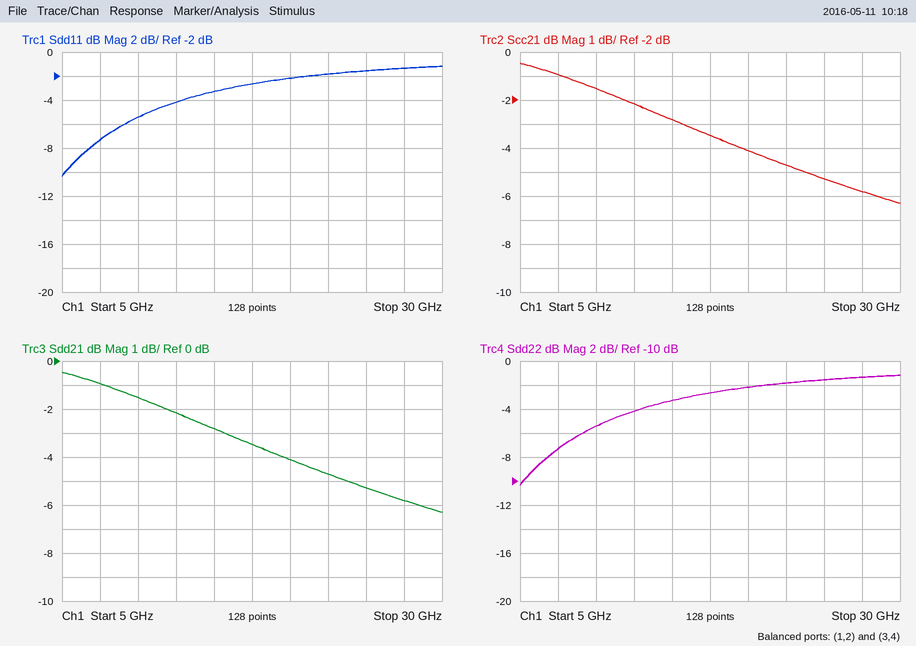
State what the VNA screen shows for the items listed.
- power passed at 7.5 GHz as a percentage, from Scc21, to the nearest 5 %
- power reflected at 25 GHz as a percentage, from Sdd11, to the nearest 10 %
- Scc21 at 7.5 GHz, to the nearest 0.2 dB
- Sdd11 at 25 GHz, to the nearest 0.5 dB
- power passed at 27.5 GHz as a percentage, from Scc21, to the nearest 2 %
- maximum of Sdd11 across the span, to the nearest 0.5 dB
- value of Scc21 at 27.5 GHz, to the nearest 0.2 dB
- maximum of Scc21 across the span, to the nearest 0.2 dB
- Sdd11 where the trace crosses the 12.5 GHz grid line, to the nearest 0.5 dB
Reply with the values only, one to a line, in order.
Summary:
80 %
70 %
-1.0 dB
-1.5 dB
26 %
-1.0 dB
-5.8 dB
-0.4 dB
-4.0 dB
